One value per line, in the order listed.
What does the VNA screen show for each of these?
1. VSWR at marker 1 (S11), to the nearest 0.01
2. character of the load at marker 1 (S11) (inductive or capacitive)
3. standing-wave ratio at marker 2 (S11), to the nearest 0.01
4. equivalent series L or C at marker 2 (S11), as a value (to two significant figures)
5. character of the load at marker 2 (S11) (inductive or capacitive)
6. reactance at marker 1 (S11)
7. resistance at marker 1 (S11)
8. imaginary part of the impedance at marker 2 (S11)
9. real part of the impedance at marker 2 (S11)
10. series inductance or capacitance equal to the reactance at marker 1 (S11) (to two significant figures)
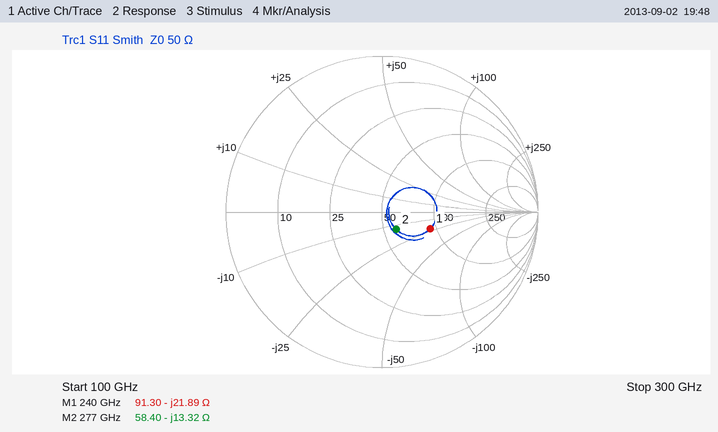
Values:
1.97
capacitive
1.34
43 fF
capacitive
-21.89 Ω
91.30 Ω
-13.32 Ω
58.40 Ω
30 fF
